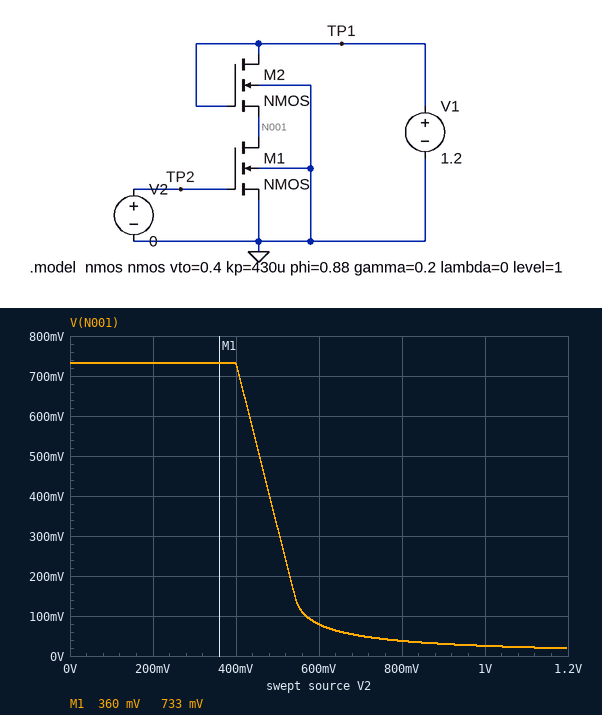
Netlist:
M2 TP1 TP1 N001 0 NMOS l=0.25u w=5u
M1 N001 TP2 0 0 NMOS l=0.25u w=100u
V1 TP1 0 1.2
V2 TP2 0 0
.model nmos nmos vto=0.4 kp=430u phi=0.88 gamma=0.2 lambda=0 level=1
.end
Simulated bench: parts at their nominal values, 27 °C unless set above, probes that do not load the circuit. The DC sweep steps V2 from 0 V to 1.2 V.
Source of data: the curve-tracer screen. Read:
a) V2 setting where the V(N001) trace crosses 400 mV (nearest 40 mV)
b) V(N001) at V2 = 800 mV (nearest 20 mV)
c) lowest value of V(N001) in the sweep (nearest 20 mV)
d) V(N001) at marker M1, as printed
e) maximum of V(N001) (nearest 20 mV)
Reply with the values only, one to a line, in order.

480 mV
40 mV
20 mV
733 mV
740 mV
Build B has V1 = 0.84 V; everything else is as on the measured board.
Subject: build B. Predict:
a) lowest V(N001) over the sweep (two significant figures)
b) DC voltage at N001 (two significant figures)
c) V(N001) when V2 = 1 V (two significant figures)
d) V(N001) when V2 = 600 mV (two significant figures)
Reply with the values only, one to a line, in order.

5.9 mV
400 mV
7.8 mV
23 mV
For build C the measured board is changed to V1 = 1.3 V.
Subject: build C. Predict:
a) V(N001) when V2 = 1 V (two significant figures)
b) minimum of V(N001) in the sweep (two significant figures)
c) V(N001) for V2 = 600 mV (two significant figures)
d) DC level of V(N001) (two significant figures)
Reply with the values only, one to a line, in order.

32 mV
24 mV
100 mV
830 mV
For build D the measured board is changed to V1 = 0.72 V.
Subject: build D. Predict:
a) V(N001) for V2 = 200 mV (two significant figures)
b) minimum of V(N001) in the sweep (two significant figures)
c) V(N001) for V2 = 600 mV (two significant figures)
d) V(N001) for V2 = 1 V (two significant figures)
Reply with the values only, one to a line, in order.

290 mV
3.1 mV
12 mV
4.2 mV
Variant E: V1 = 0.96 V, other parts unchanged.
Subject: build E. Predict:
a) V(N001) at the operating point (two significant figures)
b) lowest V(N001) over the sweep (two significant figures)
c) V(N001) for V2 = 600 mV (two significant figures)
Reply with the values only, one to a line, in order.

510 mV
9.5 mV
37 mV
